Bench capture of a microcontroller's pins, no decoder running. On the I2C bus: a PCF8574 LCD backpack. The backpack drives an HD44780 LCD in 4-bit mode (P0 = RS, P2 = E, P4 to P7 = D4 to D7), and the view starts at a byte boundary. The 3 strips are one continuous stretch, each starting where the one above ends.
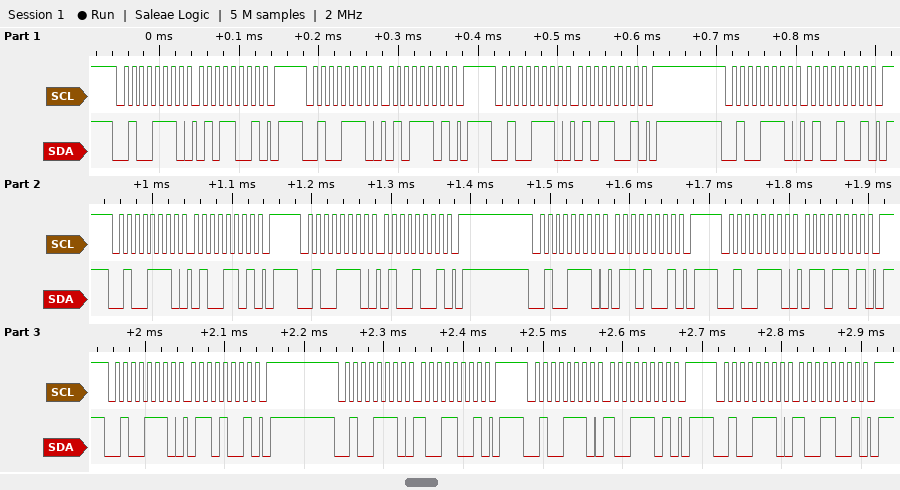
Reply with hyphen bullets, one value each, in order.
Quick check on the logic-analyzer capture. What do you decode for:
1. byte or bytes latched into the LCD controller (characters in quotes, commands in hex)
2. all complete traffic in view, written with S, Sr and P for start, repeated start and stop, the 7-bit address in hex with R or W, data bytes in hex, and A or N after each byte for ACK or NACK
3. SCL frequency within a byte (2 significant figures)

- 'T' 'i'
- S 27W A 59 A P S 27W A 5D A P S 27W A 59 A P S 27W A 49 A P S 27W A 4D A P S 27W A 49 A P S 27W A 69 A P S 27W A 6D A P S 27W A 69 A P S 27W A 99 A P S 27W A 9D A P S 27W A 99 A P
- 100 kHz
